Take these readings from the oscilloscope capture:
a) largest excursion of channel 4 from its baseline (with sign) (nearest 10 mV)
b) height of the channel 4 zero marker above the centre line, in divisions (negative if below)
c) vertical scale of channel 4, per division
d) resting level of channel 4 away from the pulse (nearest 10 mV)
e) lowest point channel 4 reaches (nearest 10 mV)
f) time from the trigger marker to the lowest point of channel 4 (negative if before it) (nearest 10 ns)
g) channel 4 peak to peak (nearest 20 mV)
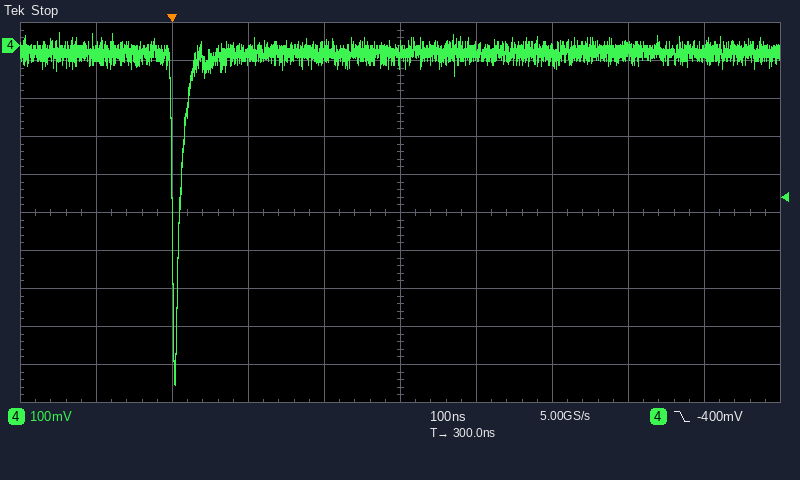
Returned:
-870 mV
+4.4 div
100 mV
-20 mV
-890 mV
0 ns
920 mV
